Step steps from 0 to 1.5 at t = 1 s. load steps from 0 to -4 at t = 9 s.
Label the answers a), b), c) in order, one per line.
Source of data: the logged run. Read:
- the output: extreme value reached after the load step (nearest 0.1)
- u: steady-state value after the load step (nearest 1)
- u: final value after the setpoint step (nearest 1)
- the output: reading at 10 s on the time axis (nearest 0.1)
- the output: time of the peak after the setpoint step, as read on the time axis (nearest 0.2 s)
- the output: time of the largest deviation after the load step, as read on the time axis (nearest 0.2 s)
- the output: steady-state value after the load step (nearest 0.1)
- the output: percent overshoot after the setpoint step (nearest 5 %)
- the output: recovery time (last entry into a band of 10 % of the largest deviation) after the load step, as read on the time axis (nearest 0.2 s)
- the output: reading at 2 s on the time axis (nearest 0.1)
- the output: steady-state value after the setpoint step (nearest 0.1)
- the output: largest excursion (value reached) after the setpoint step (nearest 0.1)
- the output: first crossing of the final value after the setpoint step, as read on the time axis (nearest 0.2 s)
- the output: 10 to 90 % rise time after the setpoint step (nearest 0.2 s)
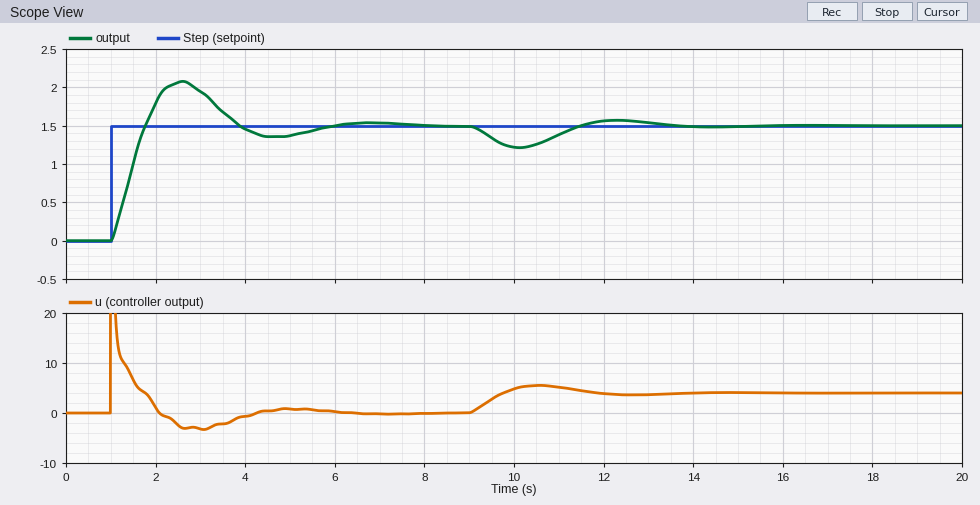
a) 1.2
b) 4
c) 0
d) 1.2
e) 2.6 s
f) 10.2 s
g) 1.5
h) 40 %
i) 13.2 s
j) 1.8
k) 1.5
l) 2.1
m) 1.8 s
n) 0.6 s
